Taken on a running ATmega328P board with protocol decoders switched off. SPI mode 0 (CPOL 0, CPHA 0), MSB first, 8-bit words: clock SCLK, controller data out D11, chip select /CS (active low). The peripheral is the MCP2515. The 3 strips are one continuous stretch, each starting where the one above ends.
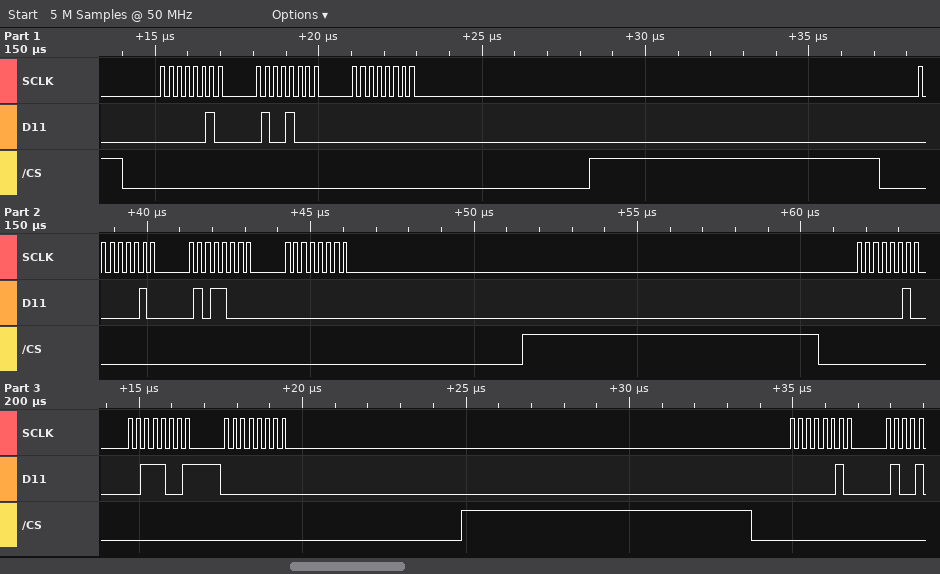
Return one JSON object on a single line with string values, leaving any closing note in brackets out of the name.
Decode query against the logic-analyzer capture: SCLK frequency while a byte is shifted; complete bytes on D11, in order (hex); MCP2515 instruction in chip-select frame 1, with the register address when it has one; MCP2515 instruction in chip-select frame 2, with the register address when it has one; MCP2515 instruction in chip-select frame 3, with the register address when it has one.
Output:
{"SCLK frequency while a byte is shifted": "4 MHz", "complete bytes on D11, in order": "02 48 00 02 58 00 02 39 00 02", "MCP2515 instruction in chip-select frame 1, with the register address when it has one": "WRITE 0x48", "MCP2515 instruction in chip-select frame 2, with the register address when it has one": "WRITE 0x58", "MCP2515 instruction in chip-select frame 3, with the register address when it has one": "WRITE 0x39"}
